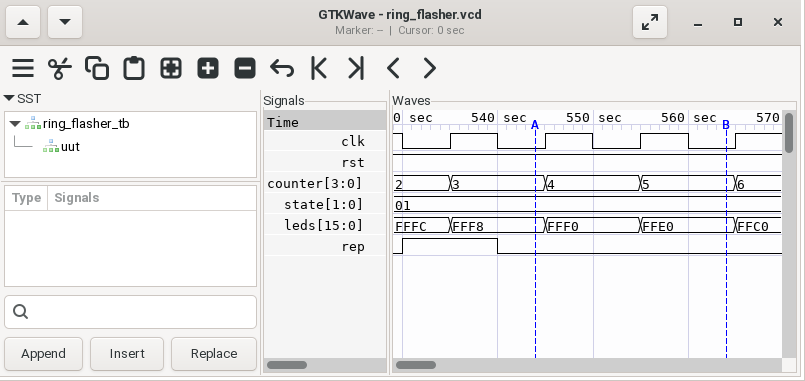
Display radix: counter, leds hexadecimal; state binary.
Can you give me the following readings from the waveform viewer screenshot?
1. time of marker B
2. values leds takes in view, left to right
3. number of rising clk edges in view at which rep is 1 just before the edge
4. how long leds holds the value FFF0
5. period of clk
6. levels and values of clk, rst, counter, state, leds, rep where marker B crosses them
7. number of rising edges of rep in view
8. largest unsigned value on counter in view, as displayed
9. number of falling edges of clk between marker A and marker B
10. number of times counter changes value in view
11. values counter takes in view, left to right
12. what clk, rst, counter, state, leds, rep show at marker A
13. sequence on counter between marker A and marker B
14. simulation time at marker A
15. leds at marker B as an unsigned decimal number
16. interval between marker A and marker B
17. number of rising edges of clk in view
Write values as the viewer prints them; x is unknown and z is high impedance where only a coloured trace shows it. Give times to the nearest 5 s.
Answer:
565 s
FFFC, FFF8, FFF0, FFE0, FFC0
1
10 s
10 s
clk=0, rst=1, counter=5, state=01, leds=FFE0, rep=0
1
6
2
4
2, 3, 4, 5, 6
clk=0, rst=1, counter=3, state=01, leds=FFF8, rep=0
3, 4, 5
545 s
65504
20 s
4
